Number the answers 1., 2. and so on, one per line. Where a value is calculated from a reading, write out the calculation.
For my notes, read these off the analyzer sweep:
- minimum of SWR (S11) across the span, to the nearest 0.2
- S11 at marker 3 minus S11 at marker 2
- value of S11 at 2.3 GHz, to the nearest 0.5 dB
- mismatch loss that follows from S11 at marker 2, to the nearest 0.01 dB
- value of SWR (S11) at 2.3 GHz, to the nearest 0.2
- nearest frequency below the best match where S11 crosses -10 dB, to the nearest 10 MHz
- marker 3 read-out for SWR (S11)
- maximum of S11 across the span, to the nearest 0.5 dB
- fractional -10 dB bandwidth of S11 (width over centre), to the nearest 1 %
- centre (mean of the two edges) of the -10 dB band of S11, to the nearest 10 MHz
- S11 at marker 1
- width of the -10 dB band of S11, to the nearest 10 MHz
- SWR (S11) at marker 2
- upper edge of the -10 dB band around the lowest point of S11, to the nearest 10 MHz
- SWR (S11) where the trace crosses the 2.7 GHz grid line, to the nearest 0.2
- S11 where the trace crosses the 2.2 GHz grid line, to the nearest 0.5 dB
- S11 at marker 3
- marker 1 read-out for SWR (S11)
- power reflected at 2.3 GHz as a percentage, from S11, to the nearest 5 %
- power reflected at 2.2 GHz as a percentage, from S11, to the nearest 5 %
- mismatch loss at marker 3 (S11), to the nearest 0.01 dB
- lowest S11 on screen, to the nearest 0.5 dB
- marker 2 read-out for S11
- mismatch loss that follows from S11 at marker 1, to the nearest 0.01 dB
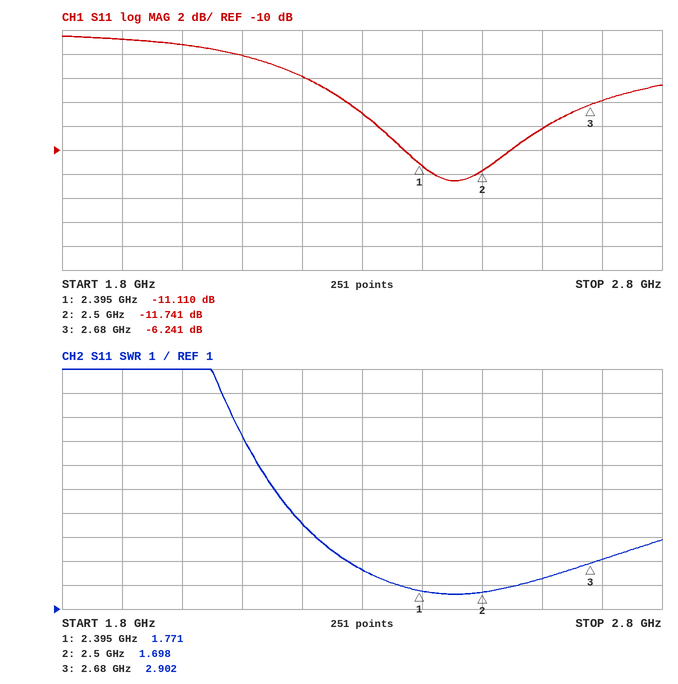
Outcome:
1. 1.6
2. -6.241 − (-11.741) = 5.500 dB
3. -7.0 dB
4. −10 log10(1 − 10^(-11.741/10)) ≈ 0.30 dB
5. 2.6
6. 2.37 GHz
7. 2.902
8. -0.5 dB
9. 180 MHz / 2.46 GHz ≈ 7 %
10. 2.46 GHz
11. -11.110 dB
12. 2.55 GHz − 2.37 GHz = 180 MHz
13. 1.698
14. 2.55 GHz
15. 3.0
16. -4.0 dB
17. -6.241 dB
18. 1.771
19. 10^(-7/10) ≈ 20 %
20. 10^(-4/10) ≈ 40 %
21. −10 log10(1 − 10^(-6.241/10)) ≈ 1.18 dB
22. -12.5 dB
23. -11.741 dB
24. −10 log10(1 − 10^(-11.11/10)) ≈ 0.35 dB
